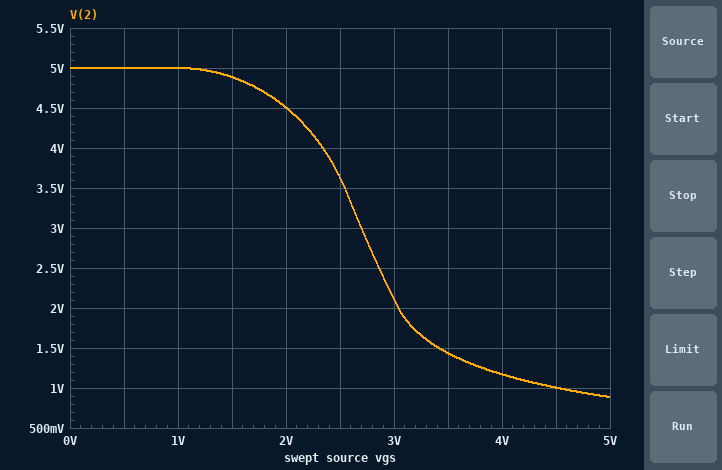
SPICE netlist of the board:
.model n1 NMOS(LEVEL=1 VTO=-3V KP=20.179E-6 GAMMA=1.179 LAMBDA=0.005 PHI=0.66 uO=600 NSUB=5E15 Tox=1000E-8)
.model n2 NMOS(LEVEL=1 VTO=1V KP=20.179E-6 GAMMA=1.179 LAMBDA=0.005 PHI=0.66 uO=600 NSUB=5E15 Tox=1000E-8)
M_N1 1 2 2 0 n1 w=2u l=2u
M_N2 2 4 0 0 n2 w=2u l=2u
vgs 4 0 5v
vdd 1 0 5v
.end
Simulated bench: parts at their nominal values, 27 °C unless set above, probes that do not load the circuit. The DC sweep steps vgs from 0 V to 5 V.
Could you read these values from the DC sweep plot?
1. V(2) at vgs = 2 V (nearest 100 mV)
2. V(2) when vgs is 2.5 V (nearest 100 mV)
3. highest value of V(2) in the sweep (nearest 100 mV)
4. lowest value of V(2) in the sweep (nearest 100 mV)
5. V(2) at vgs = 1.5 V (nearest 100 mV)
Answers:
4.5 V
3.6 V
5.0 V
900 mV
4.9 V
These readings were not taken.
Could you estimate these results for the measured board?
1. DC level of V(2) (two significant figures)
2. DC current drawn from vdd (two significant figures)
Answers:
890 mV
64 µA
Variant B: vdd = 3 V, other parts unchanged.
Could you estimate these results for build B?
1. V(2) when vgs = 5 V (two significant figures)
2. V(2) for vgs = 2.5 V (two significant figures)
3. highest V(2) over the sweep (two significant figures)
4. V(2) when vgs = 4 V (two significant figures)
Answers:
860 mV
2.3 V
3.0 V
1.1 V
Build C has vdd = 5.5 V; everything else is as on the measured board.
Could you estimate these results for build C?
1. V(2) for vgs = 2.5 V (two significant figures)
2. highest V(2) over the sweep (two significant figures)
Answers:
3.7 V
5.5 V
